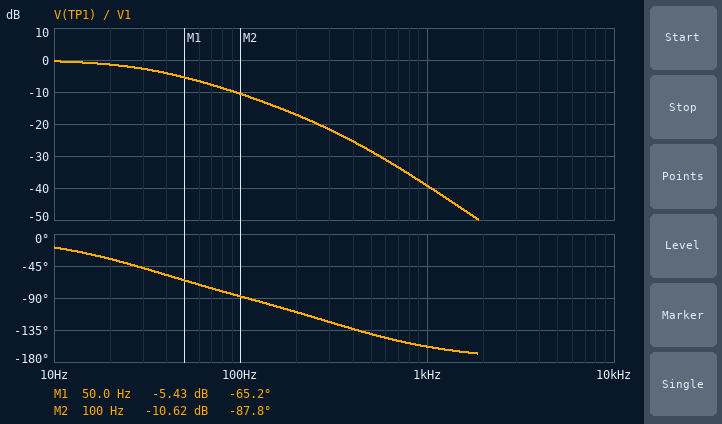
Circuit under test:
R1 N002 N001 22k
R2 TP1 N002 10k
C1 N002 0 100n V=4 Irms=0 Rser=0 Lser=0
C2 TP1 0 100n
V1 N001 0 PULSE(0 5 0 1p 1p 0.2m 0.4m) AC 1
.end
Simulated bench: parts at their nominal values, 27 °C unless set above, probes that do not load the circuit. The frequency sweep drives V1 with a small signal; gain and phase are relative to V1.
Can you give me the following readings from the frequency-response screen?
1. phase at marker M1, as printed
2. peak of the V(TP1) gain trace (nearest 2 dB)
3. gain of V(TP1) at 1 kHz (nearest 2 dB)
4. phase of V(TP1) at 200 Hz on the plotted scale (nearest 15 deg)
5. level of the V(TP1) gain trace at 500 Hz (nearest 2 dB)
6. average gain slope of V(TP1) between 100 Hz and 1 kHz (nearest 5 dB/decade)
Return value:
-65.2 deg
0 dB
-40 dB
-105 deg
-28 dB
-30 dB/decade
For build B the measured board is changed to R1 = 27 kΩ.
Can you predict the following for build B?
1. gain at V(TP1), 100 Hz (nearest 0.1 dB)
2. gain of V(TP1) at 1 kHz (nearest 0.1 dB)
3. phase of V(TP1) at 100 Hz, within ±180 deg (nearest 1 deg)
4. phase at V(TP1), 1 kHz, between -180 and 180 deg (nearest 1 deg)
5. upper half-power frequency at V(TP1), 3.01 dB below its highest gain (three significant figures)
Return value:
-12.1 dB
-41.1 dB
-91 deg
-159 deg
26.6 Hz
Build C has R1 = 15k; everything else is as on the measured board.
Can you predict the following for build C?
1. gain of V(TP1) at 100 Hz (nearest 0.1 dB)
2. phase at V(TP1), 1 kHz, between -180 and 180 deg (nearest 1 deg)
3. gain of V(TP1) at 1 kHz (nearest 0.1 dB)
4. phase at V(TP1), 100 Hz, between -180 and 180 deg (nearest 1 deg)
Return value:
-8.1 dB
-157 deg
-36.0 dB
-81 deg
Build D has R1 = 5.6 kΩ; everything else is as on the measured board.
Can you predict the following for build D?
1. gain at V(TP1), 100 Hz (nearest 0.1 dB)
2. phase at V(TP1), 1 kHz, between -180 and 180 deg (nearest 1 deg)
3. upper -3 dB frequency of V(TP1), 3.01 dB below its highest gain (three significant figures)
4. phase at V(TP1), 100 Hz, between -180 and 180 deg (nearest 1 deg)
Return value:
-3.8 dB
-148 deg
85.5 Hz
-60 deg
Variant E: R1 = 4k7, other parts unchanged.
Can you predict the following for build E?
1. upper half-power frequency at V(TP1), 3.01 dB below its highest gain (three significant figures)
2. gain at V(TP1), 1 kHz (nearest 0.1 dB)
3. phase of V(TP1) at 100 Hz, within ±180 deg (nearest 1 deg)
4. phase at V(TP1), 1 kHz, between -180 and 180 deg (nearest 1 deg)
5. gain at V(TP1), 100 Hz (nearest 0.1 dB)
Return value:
93.5 Hz
-26.6 dB
-56 deg
-145 deg
-3.3 dB
